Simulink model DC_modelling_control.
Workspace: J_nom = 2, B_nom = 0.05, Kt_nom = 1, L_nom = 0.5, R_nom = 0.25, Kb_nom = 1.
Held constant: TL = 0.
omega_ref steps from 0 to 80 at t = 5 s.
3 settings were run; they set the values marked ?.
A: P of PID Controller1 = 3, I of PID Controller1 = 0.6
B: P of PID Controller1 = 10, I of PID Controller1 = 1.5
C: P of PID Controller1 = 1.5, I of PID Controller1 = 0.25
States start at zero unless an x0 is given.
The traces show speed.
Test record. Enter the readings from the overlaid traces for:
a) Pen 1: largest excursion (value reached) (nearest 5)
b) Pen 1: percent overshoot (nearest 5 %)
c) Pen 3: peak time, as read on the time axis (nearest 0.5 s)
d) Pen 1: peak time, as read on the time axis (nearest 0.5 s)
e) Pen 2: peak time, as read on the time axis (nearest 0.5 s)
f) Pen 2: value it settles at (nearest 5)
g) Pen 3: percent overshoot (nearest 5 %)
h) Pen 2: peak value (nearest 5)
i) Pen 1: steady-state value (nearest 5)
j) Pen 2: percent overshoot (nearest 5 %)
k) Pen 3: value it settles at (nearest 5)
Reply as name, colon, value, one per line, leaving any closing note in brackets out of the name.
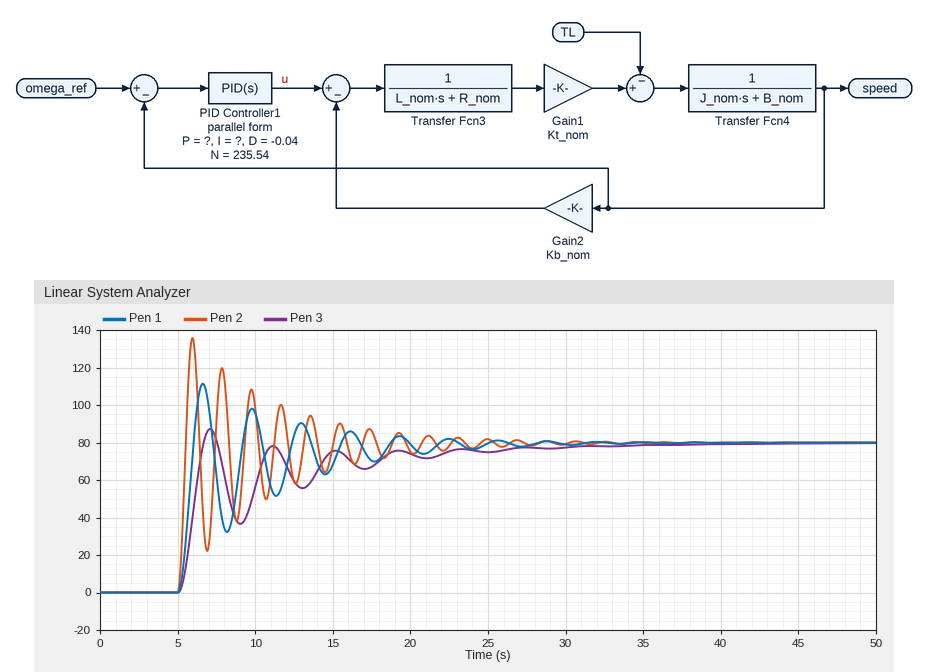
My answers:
Pen 1: largest excursion (value reached): 110
Pen 1: percent overshoot: 40 %
Pen 3: peak time, as read on the time axis: 7.0 s
Pen 1: peak time, as read on the time axis: 6.5 s
Pen 2: peak time, as read on the time axis: 6.0 s
Pen 2: value it settles at: 80
Pen 3: percent overshoot: 10 %
Pen 2: peak value: 135
Pen 1: steady-state value: 80
Pen 2: percent overshoot: 70 %
Pen 3: value it settles at: 80
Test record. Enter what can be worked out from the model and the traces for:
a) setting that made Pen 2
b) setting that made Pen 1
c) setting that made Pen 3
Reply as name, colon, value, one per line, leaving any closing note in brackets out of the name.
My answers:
setting that made Pen 2: B
setting that made Pen 1: A
setting that made Pen 3: C
